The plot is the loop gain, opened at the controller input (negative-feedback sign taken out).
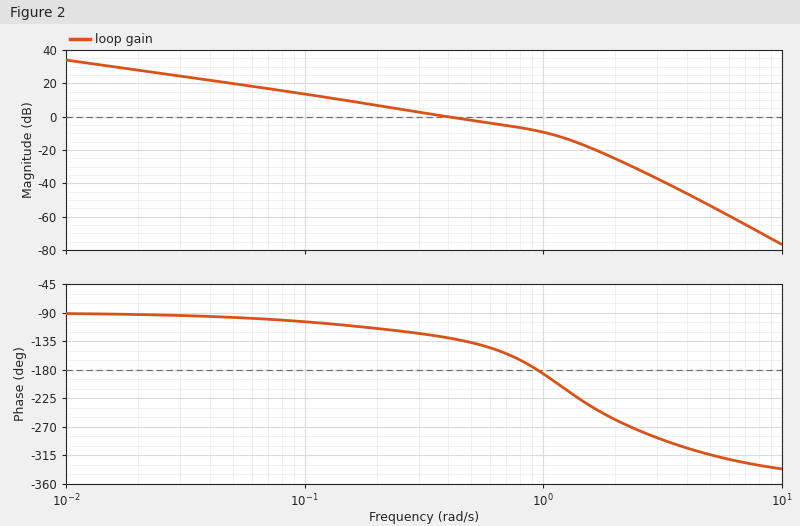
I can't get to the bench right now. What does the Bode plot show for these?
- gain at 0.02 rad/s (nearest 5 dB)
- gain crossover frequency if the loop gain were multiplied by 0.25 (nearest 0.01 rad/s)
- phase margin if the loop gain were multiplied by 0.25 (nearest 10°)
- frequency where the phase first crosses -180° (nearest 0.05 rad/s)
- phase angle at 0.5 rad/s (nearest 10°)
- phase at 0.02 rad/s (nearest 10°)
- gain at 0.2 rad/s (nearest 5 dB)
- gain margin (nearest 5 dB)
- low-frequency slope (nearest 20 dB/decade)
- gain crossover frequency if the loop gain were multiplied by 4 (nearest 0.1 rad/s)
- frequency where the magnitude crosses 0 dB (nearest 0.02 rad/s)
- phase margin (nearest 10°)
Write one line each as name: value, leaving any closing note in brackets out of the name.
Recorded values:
gain at 0.02 rad/s: 30 dB
gain crossover frequency if the loop gain were multiplied by 0.25: 0.12 rad/s
phase margin if the loop gain were multiplied by 0.25: 70°
frequency where the phase first crosses -180°: 0.95 rad/s
phase angle at 0.5 rad/s: -140°
phase at 0.02 rad/s: -90°
gain at 0.2 rad/s: 5 dB
gain margin: 10 dB
low-frequency slope: -20 dB/decade
gain crossover frequency if the loop gain were multiplied by 4: 1.2 rad/s
frequency where the magnitude crosses 0 dB: 0.40 rad/s
phase margin: 50°
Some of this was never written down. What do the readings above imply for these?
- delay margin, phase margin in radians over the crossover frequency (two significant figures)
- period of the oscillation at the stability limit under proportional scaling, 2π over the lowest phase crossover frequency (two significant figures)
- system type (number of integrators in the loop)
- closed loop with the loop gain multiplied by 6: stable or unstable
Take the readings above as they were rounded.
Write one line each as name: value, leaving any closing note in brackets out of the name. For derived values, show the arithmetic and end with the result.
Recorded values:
delay margin, phase margin in radians over the crossover frequency: 50 × π / 180 / 0.4 = 2.2 s
period of the oscillation at the stability limit under proportional scaling, 2π over the lowest phase crossover frequency: 2π / 0.95 = 6.6 s
system type: 1
closed loop with the loop gain multiplied by 6: stable or unstable: unstable
